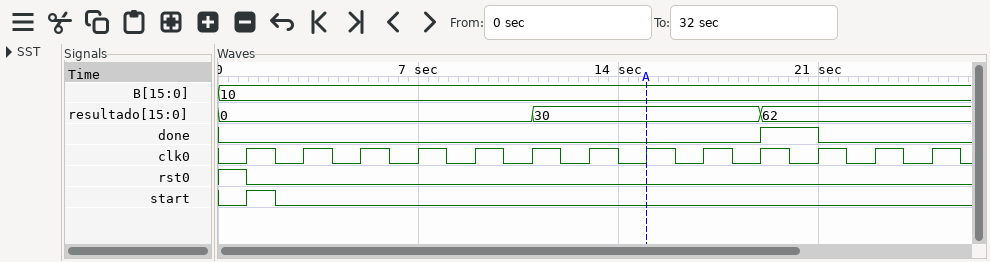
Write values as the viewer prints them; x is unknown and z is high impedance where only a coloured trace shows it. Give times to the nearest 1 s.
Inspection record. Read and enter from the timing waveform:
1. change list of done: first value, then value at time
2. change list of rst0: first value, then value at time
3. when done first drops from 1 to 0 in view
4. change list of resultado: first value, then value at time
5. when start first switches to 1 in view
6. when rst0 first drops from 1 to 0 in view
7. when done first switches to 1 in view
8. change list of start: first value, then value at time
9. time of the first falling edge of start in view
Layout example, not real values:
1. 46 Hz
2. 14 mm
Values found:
1. 0, 1 at 19 s, 0 at 21 s
2. 1, 0 at 1 s
3. 21 s
4. 0, 30 at 11 s, 62 at 19 s
5. 1 s
6. 1 s
7. 19 s
8. 0, 1 at 1 s, 0 at 2 s
9. 2 s
